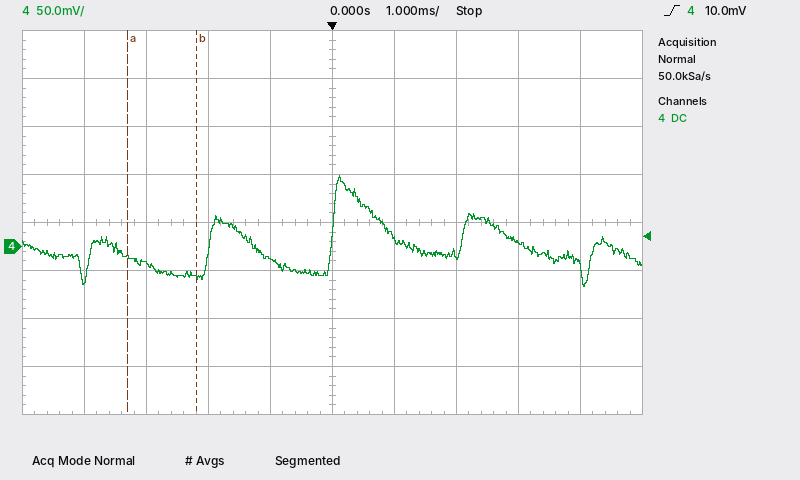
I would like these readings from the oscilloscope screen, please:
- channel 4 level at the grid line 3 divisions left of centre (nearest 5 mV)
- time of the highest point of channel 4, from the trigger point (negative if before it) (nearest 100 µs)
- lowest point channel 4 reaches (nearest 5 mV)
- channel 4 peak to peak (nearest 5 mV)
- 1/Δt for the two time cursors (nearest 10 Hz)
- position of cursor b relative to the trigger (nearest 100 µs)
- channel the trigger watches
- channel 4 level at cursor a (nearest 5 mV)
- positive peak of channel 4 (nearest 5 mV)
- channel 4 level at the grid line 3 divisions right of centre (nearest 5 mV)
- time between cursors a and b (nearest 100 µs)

-20 mV
+100 µs
-40 mV
115 mV
910 Hz
-2.2 ms
channel 4
-10 mV
75 mV
5 mV
1.1 ms
